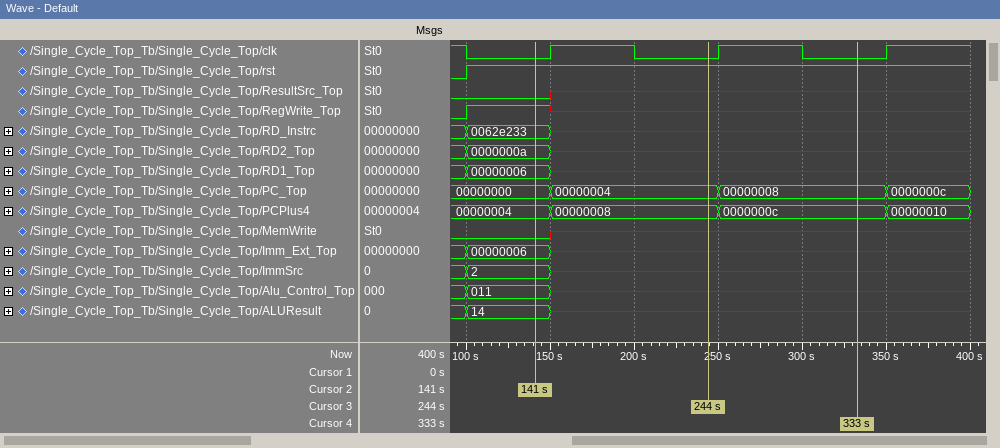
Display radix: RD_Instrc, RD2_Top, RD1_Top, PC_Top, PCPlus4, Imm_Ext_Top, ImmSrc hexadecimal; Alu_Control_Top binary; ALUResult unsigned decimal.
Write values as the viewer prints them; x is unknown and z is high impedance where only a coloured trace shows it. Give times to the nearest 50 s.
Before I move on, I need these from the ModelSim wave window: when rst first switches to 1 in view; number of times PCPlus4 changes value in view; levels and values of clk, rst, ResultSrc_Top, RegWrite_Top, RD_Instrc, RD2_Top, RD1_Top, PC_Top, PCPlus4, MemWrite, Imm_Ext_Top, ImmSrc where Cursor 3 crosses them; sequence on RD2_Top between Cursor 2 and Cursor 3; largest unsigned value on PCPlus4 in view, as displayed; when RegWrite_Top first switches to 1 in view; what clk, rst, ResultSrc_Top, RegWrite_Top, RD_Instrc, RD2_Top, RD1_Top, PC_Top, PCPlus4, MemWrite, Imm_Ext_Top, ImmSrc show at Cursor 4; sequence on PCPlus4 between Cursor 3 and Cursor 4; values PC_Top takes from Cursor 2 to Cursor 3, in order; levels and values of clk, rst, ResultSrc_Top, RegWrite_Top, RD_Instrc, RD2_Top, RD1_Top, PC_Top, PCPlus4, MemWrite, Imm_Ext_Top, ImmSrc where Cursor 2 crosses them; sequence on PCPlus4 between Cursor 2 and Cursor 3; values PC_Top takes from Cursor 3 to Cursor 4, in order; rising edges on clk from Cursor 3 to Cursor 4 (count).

100 s
3
clk=0, rst=1, ResultSrc_Top=x, RegWrite_Top=x, RD_Instrc=x, RD2_Top=x, RD1_Top=x, PC_Top=00000004, PCPlus4=00000008, MemWrite=x, Imm_Ext_Top=x, ImmSrc=x
0000000a, x
00000010
100 s
clk=0, rst=1, ResultSrc_Top=x, RegWrite_Top=x, RD_Instrc=x, RD2_Top=x, RD1_Top=x, PC_Top=00000008, PCPlus4=0000000c, MemWrite=x, Imm_Ext_Top=x, ImmSrc=x
00000008, 0000000c
00000000, 00000004
clk=0, rst=1, ResultSrc_Top=0, RegWrite_Top=1, RD_Instrc=0062e233, RD2_Top=0000000a, RD1_Top=00000006, PC_Top=00000000, PCPlus4=00000004, MemWrite=0, Imm_Ext_Top=00000006, ImmSrc=2
00000004, 00000008
00000004, 00000008
1
